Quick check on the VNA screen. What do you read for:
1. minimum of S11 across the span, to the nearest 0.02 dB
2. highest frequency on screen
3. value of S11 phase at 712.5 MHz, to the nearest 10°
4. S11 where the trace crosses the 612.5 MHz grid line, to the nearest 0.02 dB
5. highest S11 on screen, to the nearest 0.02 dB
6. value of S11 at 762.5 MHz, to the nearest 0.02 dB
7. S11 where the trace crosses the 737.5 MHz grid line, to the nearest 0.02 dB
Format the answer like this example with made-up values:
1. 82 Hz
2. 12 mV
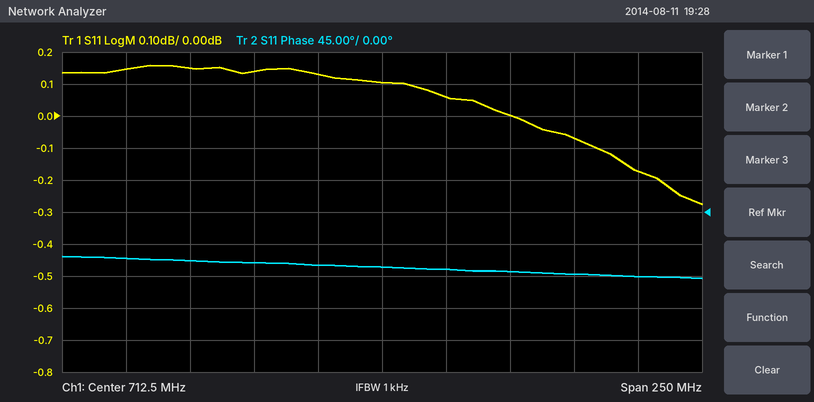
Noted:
1. -0.28 dB
2. 837.5 MHz
3. -80°
4. 0.14 dB
5. 0.16 dB
6. 0.00 dB
7. 0.06 dB
